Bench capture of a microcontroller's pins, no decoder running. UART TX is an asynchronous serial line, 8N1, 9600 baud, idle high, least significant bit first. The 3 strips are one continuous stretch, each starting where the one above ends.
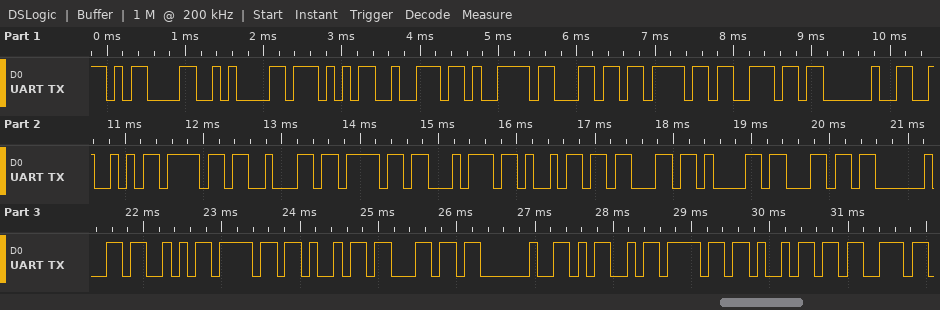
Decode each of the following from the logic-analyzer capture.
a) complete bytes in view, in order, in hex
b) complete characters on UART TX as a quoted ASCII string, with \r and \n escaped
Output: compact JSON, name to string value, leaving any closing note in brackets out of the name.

{"complete bytes in view, in order, in hex": "0D 0A 57 72 79 6C 6F 6E 20 52 6F 62 6F 74 69 63 61 6C 20 53 6F 69 6C 20 4D 6F 69 73", "complete characters on UART TX as a quoted ASCII string, with \\r and \\n escaped": "\"\\r\\nWrylon Robotical Soil Mois\""}
